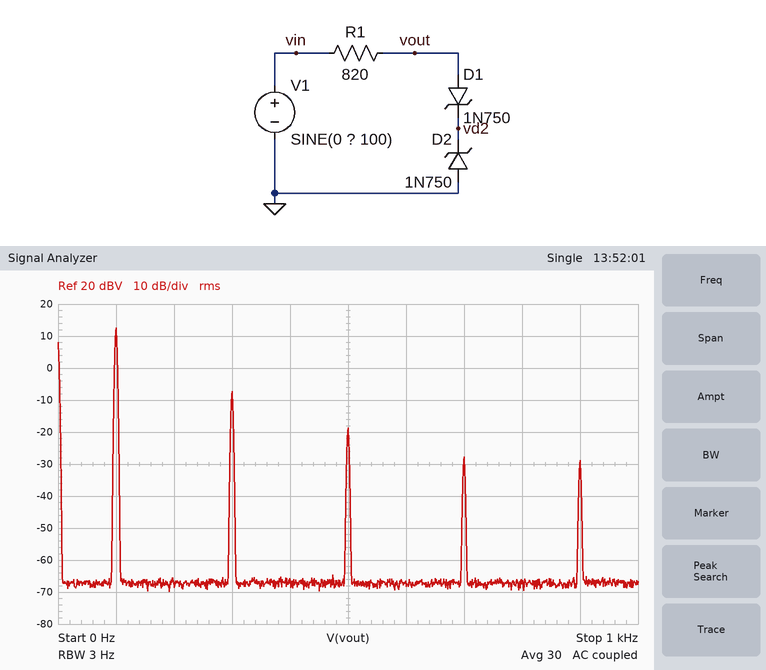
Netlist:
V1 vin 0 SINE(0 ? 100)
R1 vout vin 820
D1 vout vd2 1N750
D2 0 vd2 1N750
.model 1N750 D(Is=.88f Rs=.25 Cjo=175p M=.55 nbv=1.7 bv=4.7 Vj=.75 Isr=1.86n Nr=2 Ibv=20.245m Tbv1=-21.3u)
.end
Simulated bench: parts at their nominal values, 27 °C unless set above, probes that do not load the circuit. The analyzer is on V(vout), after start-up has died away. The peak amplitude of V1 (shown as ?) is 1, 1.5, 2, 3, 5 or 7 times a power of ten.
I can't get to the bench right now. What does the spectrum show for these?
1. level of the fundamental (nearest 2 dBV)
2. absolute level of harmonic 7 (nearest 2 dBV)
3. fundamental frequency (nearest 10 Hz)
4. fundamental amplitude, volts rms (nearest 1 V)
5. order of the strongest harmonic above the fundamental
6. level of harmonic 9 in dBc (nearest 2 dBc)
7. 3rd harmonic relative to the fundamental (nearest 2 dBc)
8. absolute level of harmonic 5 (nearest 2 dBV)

12 dBV
-28 dBV
100 Hz
4 V
3
-42 dBc
-20 dBc
-18 dBV
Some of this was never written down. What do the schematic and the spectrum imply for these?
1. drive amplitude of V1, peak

7 V
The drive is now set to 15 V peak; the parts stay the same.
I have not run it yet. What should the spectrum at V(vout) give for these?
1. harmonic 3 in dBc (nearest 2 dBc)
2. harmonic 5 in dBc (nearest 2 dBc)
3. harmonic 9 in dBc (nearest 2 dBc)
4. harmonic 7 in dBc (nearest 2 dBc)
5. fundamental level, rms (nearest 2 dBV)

-12 dBc
-20 dBc
-56 dBc
-30 dBc
14 dBV
